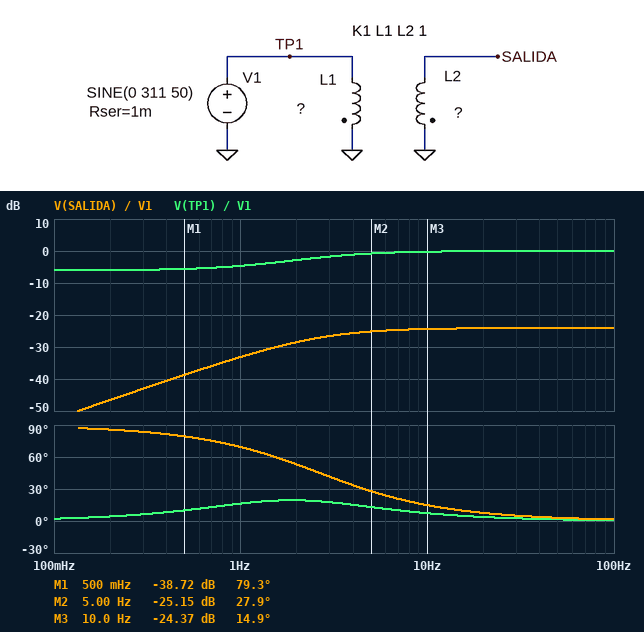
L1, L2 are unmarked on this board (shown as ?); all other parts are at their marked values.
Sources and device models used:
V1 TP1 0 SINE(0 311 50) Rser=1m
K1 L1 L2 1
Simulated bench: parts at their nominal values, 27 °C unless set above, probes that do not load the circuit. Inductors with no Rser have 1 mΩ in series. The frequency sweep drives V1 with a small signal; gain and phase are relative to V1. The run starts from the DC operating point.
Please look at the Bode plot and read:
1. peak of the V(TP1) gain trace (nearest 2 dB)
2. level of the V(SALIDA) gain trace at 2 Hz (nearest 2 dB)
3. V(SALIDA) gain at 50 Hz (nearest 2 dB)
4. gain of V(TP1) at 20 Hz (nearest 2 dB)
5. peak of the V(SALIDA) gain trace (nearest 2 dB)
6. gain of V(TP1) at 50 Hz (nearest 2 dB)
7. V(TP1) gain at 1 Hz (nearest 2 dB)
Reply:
0 dB
-28 dB
-24 dB
0 dB
-24 dB
0 dB
-4 dB
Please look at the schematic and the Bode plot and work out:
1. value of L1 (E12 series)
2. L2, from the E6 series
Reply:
120 µH
470 nH
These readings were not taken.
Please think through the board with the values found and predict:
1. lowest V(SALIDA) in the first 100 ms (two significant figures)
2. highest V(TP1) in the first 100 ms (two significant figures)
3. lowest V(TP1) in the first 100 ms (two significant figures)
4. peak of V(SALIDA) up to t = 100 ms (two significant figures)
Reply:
-20 V
310 V
-320 V
19 V
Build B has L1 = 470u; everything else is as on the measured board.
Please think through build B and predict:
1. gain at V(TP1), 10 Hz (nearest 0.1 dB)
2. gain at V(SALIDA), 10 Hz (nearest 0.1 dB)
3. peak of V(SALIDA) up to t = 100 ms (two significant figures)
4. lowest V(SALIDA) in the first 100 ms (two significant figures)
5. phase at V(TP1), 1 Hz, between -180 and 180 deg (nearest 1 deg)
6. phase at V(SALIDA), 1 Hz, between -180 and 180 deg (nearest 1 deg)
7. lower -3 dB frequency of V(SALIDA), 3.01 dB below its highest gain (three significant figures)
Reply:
0 dB
-30.0 dB
9.7 V
-10 V
15 deg
34 deg
677 mHz
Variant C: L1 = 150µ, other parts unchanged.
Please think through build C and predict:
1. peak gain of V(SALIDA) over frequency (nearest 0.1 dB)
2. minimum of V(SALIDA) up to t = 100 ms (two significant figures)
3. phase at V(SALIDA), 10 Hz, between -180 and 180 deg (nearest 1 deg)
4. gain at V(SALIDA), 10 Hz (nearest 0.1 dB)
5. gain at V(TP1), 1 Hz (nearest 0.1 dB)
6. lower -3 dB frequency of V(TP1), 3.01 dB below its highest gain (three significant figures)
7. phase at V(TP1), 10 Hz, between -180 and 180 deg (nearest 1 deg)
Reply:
-25.0 dB
-18 V
12 deg
-25.2 dB
-4.1 dB
1.50 Hz
6 deg
